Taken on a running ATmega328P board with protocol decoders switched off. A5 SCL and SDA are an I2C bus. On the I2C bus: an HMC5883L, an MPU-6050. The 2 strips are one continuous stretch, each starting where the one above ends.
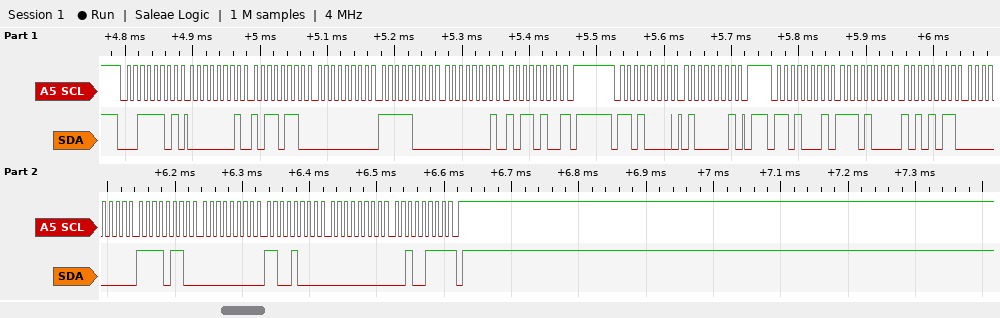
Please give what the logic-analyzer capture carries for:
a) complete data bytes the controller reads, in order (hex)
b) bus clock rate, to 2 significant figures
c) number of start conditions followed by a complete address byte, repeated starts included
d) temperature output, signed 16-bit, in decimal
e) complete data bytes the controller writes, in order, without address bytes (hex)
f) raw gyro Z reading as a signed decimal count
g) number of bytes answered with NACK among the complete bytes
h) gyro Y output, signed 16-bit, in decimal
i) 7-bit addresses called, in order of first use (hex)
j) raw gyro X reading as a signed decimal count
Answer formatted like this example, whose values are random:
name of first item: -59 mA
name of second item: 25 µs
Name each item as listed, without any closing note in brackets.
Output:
complete data bytes the controller reads, in order: 01 B6 00 F8 01 B4 E8 AB 00 F6 00 C8 00 27
bus clock rate, to 2 significant figures: 100 kHz
number of start conditions followed by a complete address byte, repeated starts included: 3
temperature output, signed 16-bit, in decimal: -5973
complete data bytes the controller writes, in order, without address bytes: 41
raw gyro Z reading as a signed decimal count: 39
number of bytes answered with NACK among the complete bytes: 2
gyro Y output, signed 16-bit, in decimal: 200
7-bit addresses called, in order of first use: 0x1E 0x68
raw gyro X reading as a signed decimal count: 246
